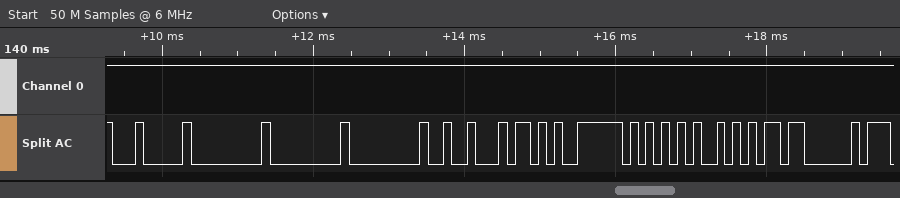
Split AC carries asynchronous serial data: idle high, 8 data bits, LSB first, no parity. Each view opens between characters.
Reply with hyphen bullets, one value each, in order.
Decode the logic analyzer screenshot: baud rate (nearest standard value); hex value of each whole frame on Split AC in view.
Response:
- 9600 baud
- 04, 00, 00, 00, 12, 2B, 55, AA, 03
